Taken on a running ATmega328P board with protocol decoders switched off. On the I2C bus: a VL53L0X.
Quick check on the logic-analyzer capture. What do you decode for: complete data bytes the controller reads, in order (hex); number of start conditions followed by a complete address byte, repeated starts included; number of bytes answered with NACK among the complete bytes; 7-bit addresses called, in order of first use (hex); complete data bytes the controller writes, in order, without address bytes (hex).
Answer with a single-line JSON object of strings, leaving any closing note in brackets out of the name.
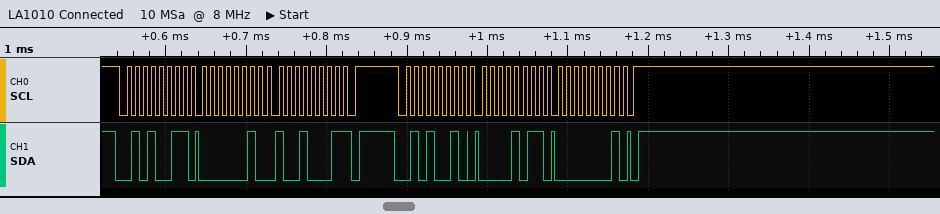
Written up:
{"complete data bytes the controller reads, in order": "02 91", "number of start conditions followed by a complete address byte, repeated starts included": "2", "number of bytes answered with NACK among the complete bytes": "1", "7-bit addresses called, in order of first use": "0x29", "complete data bytes the controller writes, in order, without address bytes": "0B 01"}
